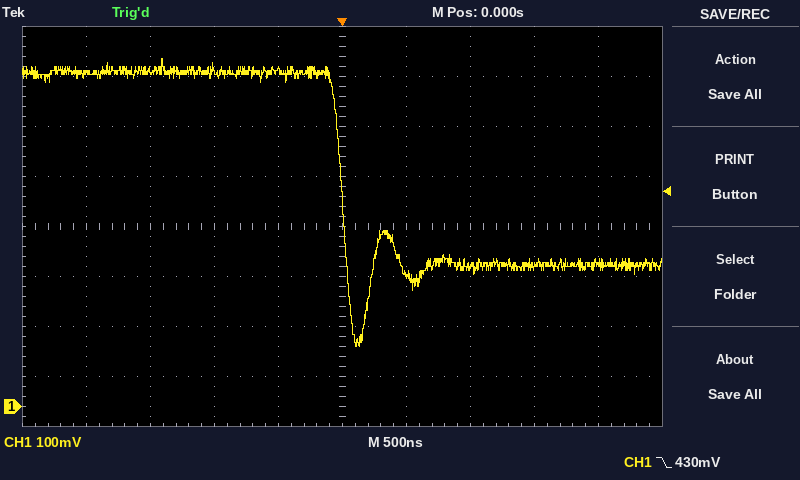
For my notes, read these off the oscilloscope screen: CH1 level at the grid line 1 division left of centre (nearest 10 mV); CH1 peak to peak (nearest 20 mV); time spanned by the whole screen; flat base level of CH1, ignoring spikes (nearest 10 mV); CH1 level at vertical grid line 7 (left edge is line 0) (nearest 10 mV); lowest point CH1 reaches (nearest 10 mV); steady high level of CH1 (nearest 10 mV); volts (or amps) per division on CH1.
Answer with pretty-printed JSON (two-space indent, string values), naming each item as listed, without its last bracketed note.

{
  "CH1 level at the grid line 1 division left of centre": "670 mV",
  "CH1 peak to peak": "580 mV",
  "time spanned by the whole screen": "5 µs",
  "flat base level of CH1, ignoring spikes": "280 mV",
  "CH1 level at vertical grid line 7 (left edge is line 0)": "280 mV",
  "lowest point CH1 reaches": "120 mV",
  "steady high level of CH1": "670 mV",
  "volts (or amps) per division on CH1": "100 mV"
}
